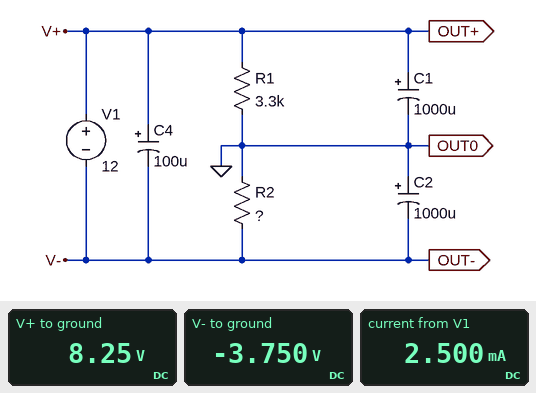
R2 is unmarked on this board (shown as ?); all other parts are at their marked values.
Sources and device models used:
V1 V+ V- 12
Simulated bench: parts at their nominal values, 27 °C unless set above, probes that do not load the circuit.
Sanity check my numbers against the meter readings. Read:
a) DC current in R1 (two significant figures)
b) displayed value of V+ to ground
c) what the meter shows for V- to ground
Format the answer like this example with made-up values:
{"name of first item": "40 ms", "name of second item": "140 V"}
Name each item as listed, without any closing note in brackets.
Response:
{"DC current in R1": "2.5 mA", "displayed value of V+ to ground": "8.25 V", "what the meter shows for V- to ground": "-3.750 V"}
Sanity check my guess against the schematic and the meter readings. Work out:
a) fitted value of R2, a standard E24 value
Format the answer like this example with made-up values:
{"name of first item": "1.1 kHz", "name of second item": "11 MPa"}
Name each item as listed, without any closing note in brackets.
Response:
{"fitted value of R2, a standard E24 value": "1.5 kΩ"}
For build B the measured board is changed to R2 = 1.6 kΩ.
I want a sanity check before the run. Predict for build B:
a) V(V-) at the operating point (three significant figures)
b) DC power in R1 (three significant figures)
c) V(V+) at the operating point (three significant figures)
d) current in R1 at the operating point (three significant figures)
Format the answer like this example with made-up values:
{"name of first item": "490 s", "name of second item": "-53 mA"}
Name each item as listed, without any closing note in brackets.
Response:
{"V(V-) at the operating point": "-3.92 V", "DC power in R1": "19.8 mW", "V(V+) at the operating point": "8.08 V", "current in R1 at the operating point": "2.45 mA"}
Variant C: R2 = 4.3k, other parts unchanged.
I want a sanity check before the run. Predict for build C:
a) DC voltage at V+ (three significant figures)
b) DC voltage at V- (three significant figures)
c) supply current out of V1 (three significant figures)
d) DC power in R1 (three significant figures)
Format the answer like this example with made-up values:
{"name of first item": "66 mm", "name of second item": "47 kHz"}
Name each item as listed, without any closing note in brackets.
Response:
{"DC voltage at V+": "5.21 V", "DC voltage at V-": "-6.79 V", "supply current out of V1": "1.58 mA", "DC power in R1": "8.23 mW"}
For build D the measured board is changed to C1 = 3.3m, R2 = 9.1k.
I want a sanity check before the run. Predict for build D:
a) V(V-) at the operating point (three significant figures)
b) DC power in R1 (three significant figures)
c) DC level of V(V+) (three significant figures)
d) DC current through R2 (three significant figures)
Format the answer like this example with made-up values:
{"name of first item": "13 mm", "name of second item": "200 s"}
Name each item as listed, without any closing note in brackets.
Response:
{"V(V-) at the operating point": "-8.81 V", "DC power in R1": "3.09 mW", "DC level of V(V+)": "3.19 V", "DC current through R2": "968 µA"}
